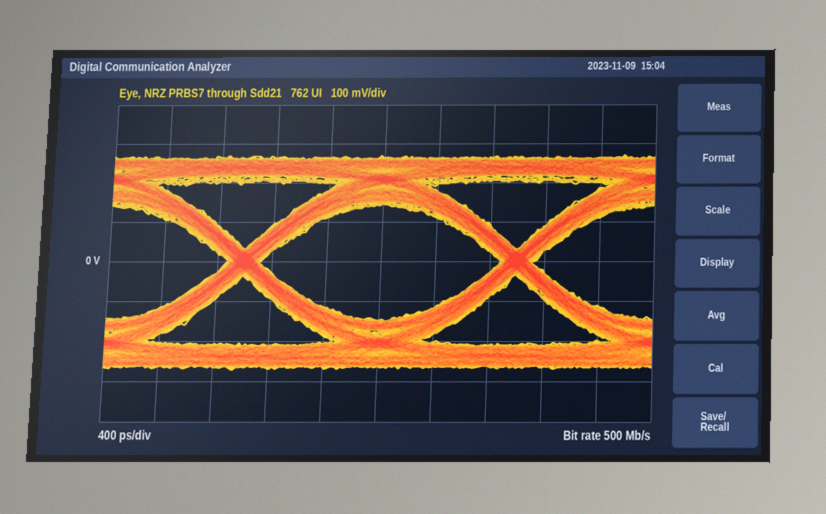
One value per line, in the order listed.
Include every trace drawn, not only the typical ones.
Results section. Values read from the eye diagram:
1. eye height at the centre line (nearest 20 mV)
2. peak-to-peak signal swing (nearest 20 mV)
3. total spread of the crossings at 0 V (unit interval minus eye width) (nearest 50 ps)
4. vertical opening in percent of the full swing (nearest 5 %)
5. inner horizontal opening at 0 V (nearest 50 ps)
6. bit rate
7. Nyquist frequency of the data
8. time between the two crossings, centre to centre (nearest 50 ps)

300 mV
540 mV
250 ps
55 %
1.75 ns
500 Mb/s
250 MHz
2.00 ns
